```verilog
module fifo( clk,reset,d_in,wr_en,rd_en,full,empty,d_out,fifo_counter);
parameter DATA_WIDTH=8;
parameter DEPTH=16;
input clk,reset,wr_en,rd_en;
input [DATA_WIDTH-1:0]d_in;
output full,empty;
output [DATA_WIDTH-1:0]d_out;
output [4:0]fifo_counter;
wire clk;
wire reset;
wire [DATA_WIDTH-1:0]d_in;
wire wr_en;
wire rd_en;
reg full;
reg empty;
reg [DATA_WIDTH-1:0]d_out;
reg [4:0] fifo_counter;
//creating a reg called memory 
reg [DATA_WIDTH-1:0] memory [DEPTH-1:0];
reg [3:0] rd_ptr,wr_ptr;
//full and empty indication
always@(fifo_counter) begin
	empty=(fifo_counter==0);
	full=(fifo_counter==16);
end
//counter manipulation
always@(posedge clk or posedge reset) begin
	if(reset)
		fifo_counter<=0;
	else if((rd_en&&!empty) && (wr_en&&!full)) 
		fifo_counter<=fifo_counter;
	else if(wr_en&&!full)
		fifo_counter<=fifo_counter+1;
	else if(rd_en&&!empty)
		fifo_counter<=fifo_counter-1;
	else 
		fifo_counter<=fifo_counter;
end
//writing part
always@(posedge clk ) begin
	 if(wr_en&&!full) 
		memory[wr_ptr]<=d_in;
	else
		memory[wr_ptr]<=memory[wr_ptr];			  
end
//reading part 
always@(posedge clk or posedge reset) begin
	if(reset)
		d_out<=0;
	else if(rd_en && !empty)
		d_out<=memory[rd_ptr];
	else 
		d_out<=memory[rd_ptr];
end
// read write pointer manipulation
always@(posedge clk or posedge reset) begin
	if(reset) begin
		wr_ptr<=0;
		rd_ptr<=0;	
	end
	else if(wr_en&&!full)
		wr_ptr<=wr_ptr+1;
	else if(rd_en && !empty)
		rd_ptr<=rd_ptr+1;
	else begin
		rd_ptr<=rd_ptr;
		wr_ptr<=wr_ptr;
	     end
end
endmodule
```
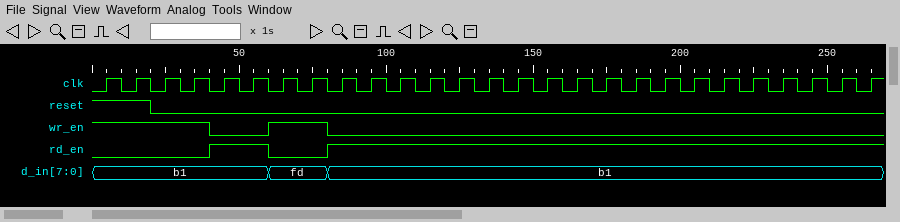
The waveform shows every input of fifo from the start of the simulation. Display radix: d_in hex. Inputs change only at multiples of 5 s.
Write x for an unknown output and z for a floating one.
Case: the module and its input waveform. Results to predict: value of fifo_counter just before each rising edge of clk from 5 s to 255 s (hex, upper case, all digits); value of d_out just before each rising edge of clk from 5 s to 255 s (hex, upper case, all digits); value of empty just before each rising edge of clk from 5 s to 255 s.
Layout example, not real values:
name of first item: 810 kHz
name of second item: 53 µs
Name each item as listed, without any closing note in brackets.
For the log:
value of fifo_counter just before each rising edge of clk from 5 s to 255 s: 00, 00, 00, 01, 02, 01, 00, 01, 02, 01, 00, 00, 00, 00, 00, 00, 00, 00, 00, 00, 00, 00, 00, 00, 00, 00
value of d_out just before each rising edge of clk from 5 s to 255 s: 00, 00, 00, B1, B1, B1, B1, x, FD, FD, FD, x, x, x, x, x, x, x, x, x, x, x, x, x, x, x
value of empty just before each rising edge of clk from 5 s to 255 s: 1 1 1 0 0 0 1 0 0 0 1 1 1 1 1 1 1 1 1 1 1 1 1 1 1 1
